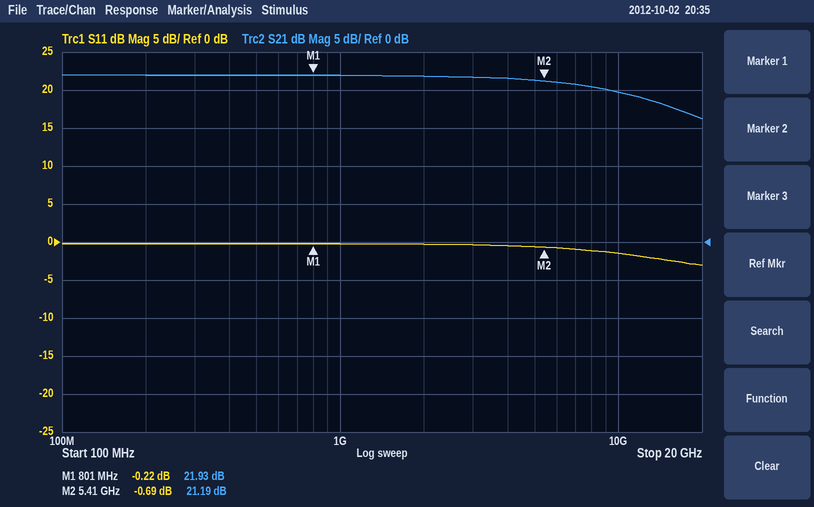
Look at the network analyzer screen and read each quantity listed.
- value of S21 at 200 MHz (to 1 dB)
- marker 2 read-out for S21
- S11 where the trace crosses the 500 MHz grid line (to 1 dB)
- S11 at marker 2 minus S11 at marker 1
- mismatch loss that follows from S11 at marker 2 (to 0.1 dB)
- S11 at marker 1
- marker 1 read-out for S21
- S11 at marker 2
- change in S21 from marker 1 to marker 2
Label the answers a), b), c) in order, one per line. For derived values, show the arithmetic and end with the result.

a) 22 dB
b) 21.19 dB
c) 0 dB
d) -0.69 − (-0.22) = -0.47 dB
e) −10 log10(1 − 10^(-0.69/10)) ≈ 8.3 dB
f) -0.22 dB
g) 21.93 dB
h) -0.69 dB
i) 21.19 − (21.93) = -0.74 dB
